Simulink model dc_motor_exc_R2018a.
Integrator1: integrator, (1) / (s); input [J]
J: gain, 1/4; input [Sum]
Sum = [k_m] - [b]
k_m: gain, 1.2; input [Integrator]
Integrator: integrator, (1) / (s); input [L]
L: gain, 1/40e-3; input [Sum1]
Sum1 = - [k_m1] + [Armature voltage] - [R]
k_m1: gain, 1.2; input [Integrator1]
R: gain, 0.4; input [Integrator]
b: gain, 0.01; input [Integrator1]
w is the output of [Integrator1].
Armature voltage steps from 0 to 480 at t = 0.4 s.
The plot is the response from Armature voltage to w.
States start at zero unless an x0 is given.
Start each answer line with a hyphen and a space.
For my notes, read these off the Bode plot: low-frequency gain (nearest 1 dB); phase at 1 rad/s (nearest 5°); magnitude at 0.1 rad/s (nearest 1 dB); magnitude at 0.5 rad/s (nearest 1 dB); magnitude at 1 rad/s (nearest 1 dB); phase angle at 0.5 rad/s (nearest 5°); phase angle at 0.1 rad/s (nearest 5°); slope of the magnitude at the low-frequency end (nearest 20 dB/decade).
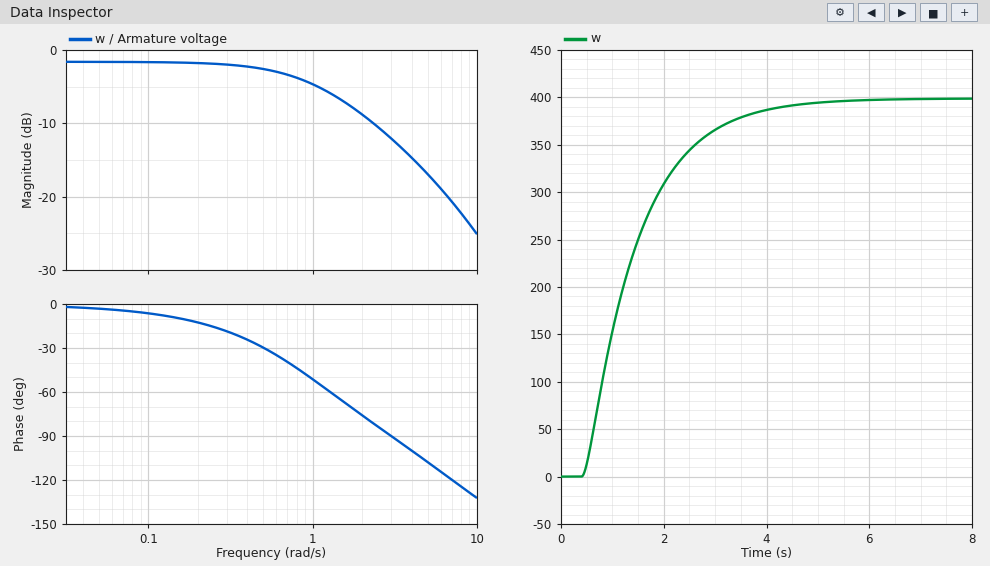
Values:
- -2 dB
- -50°
- -2 dB
- -3 dB
- -5 dB
- -30°
- -5°
- 0 dB/decade
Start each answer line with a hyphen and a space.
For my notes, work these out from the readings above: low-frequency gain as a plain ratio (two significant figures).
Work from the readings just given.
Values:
- 0.79
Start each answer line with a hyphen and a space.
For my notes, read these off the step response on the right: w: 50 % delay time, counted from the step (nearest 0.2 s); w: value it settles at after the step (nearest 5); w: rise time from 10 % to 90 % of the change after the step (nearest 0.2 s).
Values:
- 0.8 s
- 400
- 2.2 s
